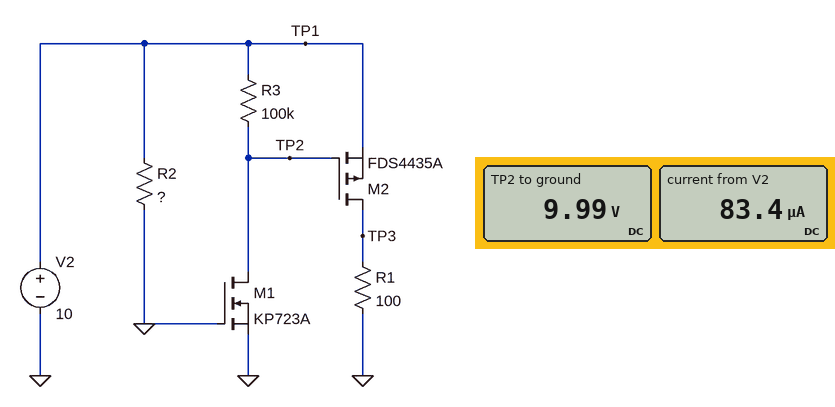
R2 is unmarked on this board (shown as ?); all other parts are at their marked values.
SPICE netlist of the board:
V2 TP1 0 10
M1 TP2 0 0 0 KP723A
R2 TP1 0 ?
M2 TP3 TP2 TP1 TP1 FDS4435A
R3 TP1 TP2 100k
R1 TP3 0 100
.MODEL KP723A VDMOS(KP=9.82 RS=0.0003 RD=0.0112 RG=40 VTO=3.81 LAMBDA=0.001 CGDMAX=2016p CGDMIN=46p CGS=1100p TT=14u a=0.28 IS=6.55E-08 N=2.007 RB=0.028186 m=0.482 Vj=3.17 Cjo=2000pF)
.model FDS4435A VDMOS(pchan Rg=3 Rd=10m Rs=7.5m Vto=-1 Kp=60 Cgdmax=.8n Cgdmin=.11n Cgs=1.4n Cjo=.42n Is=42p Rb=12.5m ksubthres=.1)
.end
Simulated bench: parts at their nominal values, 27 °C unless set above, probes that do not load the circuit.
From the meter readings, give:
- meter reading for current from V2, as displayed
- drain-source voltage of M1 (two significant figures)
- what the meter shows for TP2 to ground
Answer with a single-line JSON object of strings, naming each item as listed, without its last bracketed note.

{"meter reading for current from V2, as displayed": "83.4 µA", "drain-source voltage of M1": "10 V", "what the meter shows for TP2 to ground": "9.99 V"}
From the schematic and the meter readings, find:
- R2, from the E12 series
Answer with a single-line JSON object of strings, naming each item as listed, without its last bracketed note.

{"R2, from the E12 series": "120 kΩ"}
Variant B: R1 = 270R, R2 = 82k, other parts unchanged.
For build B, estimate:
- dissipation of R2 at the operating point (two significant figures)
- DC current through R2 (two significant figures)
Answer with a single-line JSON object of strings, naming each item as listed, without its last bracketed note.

{"dissipation of R2 at the operating point": "1.2 mW", "DC current through R2": "120 µA"}
